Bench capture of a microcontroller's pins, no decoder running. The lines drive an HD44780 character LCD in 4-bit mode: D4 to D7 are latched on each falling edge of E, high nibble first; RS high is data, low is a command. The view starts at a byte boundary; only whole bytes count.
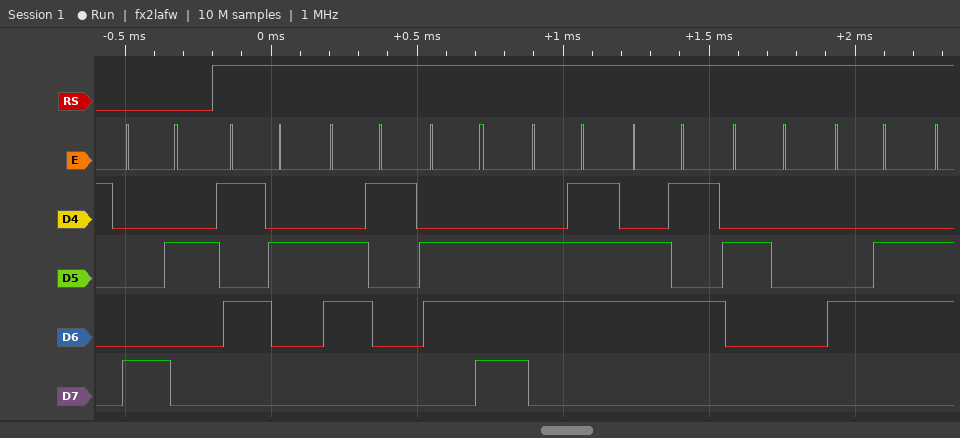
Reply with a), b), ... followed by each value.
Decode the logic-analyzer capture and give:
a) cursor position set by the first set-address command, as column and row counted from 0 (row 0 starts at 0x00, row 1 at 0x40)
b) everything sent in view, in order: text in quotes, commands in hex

a) column 2, row 0
b) 0x82 "Range F"
